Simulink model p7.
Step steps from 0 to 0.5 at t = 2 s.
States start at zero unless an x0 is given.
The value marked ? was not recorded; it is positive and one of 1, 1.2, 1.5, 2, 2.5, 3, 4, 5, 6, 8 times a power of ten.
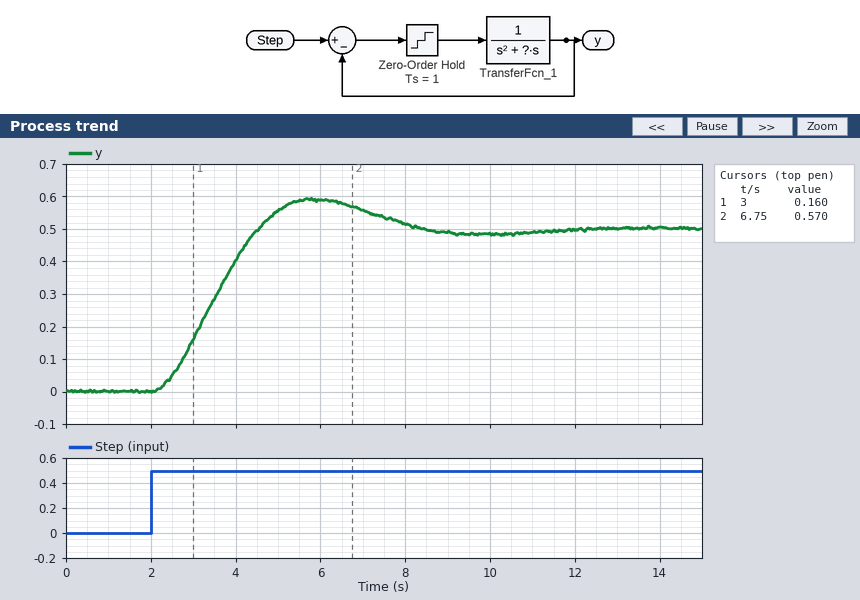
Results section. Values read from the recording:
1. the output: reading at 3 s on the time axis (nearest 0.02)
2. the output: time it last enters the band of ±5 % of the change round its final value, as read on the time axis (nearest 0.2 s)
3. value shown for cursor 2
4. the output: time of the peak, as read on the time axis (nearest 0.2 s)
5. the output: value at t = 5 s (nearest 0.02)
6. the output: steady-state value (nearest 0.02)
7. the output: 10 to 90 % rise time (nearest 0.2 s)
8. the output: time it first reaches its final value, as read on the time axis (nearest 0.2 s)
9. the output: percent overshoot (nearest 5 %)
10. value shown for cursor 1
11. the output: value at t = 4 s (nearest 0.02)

0.16
7.8 s
0.570
5.8 s
0.56
0.50
1.8 s
4.6 s
20 %
0.160
0.40
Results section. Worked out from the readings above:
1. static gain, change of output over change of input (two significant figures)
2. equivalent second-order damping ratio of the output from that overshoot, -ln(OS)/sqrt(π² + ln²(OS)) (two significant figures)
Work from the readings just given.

1.0
0.46
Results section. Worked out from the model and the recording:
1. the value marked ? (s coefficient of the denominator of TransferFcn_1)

1.5
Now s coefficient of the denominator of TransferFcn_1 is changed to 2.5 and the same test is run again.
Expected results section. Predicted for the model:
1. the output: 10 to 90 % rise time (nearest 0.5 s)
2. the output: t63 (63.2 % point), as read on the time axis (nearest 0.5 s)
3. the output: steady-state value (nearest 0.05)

3.5 s
4.0 s
0.50
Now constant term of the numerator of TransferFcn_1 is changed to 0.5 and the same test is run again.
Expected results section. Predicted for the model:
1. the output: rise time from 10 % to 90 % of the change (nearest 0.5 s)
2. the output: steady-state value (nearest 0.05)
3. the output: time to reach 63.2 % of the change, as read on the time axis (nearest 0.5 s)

4.0 s
0.50
5.0 s
